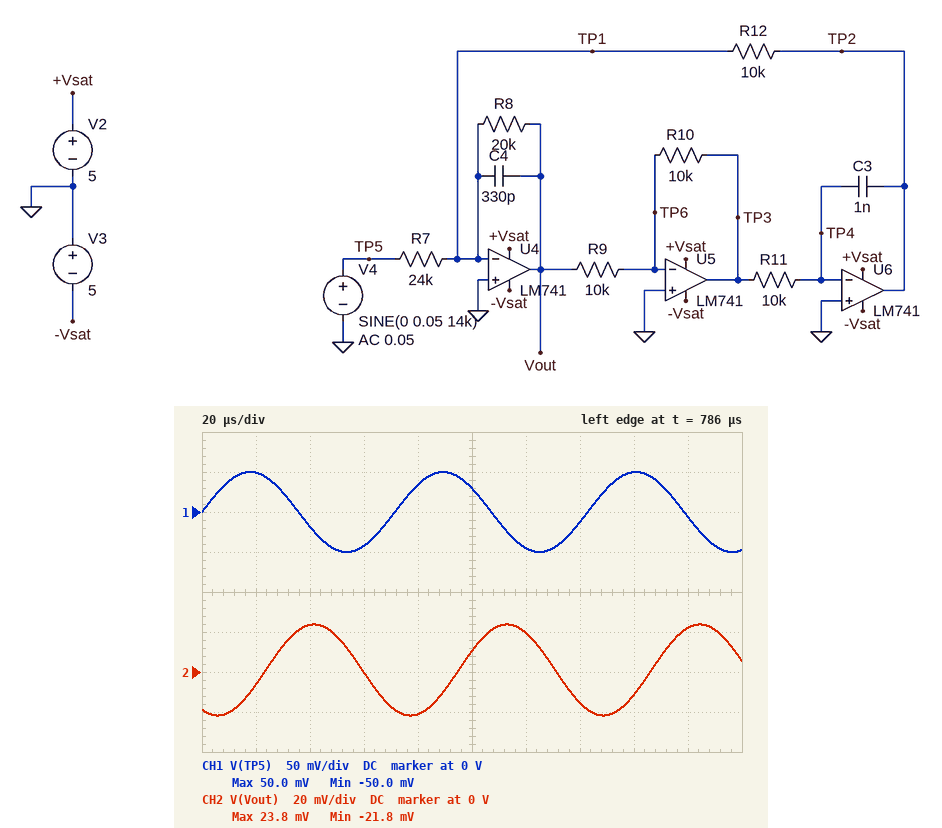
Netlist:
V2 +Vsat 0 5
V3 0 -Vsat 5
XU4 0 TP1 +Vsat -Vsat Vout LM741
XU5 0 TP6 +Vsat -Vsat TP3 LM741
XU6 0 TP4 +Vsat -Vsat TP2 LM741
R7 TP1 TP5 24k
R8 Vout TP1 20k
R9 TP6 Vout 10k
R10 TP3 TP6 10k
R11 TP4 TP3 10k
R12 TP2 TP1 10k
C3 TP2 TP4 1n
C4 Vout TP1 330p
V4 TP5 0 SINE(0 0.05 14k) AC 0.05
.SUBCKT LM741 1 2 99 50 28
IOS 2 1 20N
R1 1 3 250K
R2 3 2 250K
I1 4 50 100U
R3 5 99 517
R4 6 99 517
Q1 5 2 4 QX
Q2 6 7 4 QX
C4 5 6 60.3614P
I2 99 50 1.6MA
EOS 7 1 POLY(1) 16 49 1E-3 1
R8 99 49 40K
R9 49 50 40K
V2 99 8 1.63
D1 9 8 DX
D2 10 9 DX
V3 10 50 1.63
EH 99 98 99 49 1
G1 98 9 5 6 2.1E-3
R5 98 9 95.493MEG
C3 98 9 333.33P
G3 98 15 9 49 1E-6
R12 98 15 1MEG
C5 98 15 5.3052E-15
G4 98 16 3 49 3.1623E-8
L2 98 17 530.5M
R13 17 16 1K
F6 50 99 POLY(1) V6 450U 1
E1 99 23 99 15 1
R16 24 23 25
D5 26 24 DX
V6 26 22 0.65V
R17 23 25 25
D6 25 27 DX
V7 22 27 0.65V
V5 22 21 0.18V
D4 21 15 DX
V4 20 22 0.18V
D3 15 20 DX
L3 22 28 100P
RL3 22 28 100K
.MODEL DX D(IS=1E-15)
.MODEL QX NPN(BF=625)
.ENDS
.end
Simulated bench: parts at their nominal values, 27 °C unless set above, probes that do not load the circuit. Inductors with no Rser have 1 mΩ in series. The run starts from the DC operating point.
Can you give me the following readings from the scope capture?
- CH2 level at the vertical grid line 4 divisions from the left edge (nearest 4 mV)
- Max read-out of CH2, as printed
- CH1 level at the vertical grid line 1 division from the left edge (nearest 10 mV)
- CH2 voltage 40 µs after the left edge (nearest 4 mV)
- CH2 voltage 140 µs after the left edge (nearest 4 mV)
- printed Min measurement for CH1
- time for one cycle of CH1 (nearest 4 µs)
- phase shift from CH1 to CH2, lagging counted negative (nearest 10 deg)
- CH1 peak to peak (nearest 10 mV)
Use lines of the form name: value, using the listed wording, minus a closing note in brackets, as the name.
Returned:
CH2 level at the vertical grid line 4 divisions from the left edge: -20 mV
Max read-out of CH2, as printed: 23.8 mV
CH1 level at the vertical grid line 1 division from the left edge: 50 mV
CH2 voltage 40 µs after the left edge: 24 mV
CH2 voltage 140 µs after the left edge: -16 mV
printed Min measurement for CH1: -50.0 mV
time for one cycle of CH1: 72 µs
phase shift from CH1 to CH2, lagging counted negative: -120 deg
CH1 peak to peak: 100 mV
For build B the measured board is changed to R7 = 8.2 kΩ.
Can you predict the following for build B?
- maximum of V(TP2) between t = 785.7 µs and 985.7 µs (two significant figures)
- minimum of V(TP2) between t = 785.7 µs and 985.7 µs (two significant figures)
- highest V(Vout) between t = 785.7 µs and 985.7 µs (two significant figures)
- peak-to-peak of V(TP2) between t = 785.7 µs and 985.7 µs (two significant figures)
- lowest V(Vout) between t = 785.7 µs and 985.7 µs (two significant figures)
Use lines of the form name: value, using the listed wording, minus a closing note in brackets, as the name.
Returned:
maximum of V(TP2) between t = 785.7 µs and 985.7 µs: 79 mV
minimum of V(TP2) between t = 785.7 µs and 985.7 µs: -72 mV
highest V(Vout) between t = 785.7 µs and 985.7 µs: 68 mV
peak-to-peak of V(TP2) between t = 785.7 µs and 985.7 µs: 150 mV
lowest V(Vout) between t = 785.7 µs and 985.7 µs: -66 mV
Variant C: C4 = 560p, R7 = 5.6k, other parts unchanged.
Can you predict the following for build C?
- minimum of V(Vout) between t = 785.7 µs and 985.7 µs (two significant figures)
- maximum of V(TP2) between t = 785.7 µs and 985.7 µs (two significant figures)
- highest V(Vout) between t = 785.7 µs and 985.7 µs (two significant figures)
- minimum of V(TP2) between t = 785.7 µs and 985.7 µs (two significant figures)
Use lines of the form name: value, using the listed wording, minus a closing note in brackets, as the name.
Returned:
minimum of V(Vout) between t = 785.7 µs and 985.7 µs: -120 mV
maximum of V(TP2) between t = 785.7 µs and 985.7 µs: 140 mV
highest V(Vout) between t = 785.7 µs and 985.7 µs: 120 mV
minimum of V(TP2) between t = 785.7 µs and 985.7 µs: -130 mV
